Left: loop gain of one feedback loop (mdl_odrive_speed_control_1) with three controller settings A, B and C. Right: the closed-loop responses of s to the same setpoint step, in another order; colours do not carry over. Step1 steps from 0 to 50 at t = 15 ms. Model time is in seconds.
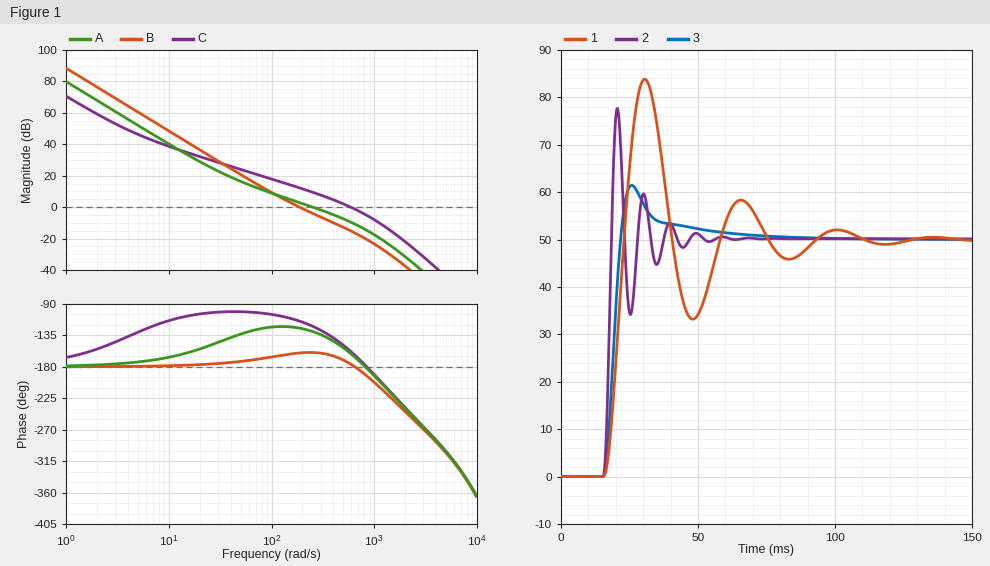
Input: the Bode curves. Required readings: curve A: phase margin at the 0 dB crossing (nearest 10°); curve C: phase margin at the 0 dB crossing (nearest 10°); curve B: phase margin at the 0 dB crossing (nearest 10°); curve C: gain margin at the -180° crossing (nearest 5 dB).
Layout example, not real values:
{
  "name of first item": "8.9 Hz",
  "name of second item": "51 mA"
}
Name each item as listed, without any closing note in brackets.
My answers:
{
  "curve A: phase margin at the 0 dB crossing": "50°",
  "curve C: phase margin at the 0 dB crossing": "20°",
  "curve B: phase margin at the 0 dB crossing": "20°",
  "curve C: gain margin at the -180° crossing": "5 dB"
}
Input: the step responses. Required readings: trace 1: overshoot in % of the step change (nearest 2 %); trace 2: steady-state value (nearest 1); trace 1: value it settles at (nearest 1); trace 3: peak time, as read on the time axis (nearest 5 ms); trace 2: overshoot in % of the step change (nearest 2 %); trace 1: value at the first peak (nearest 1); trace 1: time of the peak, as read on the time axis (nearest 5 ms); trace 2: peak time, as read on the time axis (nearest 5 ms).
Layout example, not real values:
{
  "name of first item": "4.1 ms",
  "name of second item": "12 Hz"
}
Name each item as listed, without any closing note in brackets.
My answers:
{
  "trace 1: overshoot in % of the step change": "68 %",
  "trace 2: steady-state value": "50",
  "trace 1: value it settles at": "50",
  "trace 3: peak time, as read on the time axis": "25 ms",
  "trace 2: overshoot in % of the step change": "56 %",
  "trace 1: value at the first peak": "84",
  "trace 1: time of the peak, as read on the time axis": "30 ms",
  "trace 2: peak time, as read on the time axis": "20 ms"
}
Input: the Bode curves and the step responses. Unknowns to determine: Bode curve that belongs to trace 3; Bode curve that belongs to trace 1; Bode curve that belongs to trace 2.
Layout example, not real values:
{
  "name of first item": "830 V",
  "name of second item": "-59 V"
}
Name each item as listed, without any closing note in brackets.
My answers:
{
  "Bode curve that belongs to trace 3": "A",
  "Bode curve that belongs to trace 1": "B",
  "Bode curve that belongs to trace 2": "C"
}
